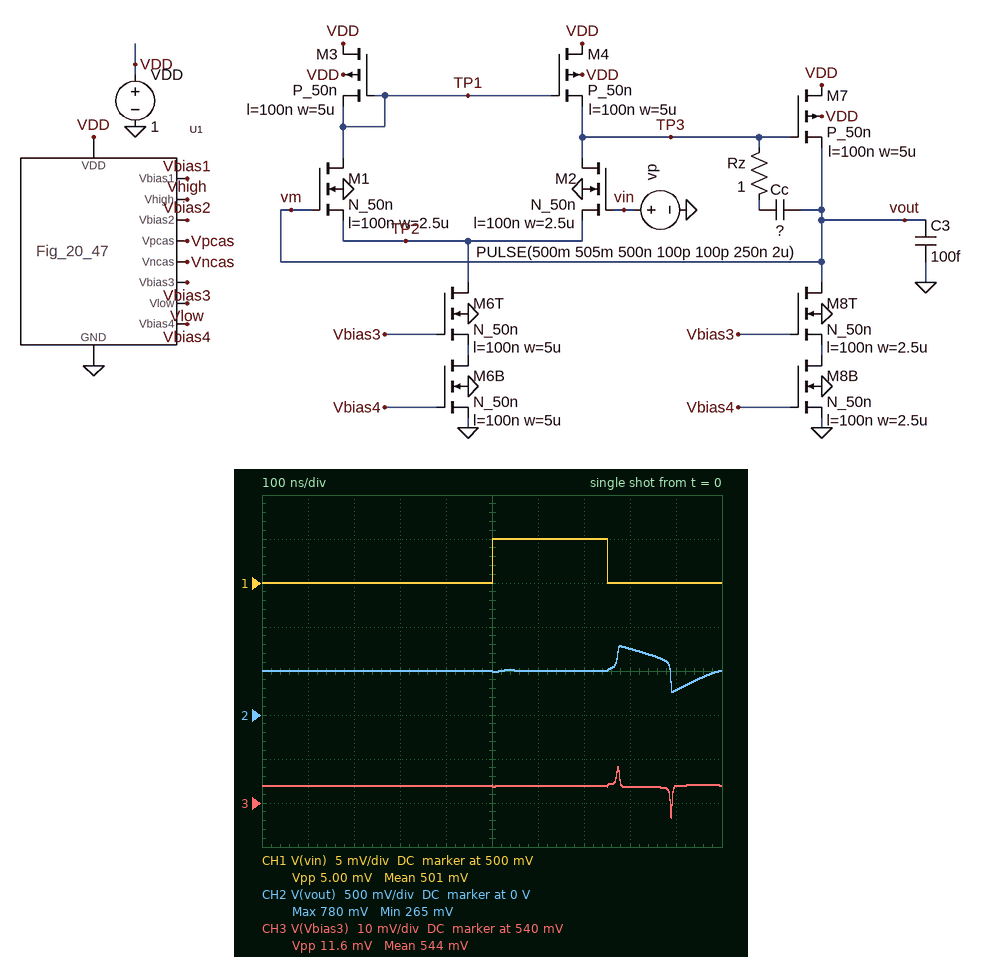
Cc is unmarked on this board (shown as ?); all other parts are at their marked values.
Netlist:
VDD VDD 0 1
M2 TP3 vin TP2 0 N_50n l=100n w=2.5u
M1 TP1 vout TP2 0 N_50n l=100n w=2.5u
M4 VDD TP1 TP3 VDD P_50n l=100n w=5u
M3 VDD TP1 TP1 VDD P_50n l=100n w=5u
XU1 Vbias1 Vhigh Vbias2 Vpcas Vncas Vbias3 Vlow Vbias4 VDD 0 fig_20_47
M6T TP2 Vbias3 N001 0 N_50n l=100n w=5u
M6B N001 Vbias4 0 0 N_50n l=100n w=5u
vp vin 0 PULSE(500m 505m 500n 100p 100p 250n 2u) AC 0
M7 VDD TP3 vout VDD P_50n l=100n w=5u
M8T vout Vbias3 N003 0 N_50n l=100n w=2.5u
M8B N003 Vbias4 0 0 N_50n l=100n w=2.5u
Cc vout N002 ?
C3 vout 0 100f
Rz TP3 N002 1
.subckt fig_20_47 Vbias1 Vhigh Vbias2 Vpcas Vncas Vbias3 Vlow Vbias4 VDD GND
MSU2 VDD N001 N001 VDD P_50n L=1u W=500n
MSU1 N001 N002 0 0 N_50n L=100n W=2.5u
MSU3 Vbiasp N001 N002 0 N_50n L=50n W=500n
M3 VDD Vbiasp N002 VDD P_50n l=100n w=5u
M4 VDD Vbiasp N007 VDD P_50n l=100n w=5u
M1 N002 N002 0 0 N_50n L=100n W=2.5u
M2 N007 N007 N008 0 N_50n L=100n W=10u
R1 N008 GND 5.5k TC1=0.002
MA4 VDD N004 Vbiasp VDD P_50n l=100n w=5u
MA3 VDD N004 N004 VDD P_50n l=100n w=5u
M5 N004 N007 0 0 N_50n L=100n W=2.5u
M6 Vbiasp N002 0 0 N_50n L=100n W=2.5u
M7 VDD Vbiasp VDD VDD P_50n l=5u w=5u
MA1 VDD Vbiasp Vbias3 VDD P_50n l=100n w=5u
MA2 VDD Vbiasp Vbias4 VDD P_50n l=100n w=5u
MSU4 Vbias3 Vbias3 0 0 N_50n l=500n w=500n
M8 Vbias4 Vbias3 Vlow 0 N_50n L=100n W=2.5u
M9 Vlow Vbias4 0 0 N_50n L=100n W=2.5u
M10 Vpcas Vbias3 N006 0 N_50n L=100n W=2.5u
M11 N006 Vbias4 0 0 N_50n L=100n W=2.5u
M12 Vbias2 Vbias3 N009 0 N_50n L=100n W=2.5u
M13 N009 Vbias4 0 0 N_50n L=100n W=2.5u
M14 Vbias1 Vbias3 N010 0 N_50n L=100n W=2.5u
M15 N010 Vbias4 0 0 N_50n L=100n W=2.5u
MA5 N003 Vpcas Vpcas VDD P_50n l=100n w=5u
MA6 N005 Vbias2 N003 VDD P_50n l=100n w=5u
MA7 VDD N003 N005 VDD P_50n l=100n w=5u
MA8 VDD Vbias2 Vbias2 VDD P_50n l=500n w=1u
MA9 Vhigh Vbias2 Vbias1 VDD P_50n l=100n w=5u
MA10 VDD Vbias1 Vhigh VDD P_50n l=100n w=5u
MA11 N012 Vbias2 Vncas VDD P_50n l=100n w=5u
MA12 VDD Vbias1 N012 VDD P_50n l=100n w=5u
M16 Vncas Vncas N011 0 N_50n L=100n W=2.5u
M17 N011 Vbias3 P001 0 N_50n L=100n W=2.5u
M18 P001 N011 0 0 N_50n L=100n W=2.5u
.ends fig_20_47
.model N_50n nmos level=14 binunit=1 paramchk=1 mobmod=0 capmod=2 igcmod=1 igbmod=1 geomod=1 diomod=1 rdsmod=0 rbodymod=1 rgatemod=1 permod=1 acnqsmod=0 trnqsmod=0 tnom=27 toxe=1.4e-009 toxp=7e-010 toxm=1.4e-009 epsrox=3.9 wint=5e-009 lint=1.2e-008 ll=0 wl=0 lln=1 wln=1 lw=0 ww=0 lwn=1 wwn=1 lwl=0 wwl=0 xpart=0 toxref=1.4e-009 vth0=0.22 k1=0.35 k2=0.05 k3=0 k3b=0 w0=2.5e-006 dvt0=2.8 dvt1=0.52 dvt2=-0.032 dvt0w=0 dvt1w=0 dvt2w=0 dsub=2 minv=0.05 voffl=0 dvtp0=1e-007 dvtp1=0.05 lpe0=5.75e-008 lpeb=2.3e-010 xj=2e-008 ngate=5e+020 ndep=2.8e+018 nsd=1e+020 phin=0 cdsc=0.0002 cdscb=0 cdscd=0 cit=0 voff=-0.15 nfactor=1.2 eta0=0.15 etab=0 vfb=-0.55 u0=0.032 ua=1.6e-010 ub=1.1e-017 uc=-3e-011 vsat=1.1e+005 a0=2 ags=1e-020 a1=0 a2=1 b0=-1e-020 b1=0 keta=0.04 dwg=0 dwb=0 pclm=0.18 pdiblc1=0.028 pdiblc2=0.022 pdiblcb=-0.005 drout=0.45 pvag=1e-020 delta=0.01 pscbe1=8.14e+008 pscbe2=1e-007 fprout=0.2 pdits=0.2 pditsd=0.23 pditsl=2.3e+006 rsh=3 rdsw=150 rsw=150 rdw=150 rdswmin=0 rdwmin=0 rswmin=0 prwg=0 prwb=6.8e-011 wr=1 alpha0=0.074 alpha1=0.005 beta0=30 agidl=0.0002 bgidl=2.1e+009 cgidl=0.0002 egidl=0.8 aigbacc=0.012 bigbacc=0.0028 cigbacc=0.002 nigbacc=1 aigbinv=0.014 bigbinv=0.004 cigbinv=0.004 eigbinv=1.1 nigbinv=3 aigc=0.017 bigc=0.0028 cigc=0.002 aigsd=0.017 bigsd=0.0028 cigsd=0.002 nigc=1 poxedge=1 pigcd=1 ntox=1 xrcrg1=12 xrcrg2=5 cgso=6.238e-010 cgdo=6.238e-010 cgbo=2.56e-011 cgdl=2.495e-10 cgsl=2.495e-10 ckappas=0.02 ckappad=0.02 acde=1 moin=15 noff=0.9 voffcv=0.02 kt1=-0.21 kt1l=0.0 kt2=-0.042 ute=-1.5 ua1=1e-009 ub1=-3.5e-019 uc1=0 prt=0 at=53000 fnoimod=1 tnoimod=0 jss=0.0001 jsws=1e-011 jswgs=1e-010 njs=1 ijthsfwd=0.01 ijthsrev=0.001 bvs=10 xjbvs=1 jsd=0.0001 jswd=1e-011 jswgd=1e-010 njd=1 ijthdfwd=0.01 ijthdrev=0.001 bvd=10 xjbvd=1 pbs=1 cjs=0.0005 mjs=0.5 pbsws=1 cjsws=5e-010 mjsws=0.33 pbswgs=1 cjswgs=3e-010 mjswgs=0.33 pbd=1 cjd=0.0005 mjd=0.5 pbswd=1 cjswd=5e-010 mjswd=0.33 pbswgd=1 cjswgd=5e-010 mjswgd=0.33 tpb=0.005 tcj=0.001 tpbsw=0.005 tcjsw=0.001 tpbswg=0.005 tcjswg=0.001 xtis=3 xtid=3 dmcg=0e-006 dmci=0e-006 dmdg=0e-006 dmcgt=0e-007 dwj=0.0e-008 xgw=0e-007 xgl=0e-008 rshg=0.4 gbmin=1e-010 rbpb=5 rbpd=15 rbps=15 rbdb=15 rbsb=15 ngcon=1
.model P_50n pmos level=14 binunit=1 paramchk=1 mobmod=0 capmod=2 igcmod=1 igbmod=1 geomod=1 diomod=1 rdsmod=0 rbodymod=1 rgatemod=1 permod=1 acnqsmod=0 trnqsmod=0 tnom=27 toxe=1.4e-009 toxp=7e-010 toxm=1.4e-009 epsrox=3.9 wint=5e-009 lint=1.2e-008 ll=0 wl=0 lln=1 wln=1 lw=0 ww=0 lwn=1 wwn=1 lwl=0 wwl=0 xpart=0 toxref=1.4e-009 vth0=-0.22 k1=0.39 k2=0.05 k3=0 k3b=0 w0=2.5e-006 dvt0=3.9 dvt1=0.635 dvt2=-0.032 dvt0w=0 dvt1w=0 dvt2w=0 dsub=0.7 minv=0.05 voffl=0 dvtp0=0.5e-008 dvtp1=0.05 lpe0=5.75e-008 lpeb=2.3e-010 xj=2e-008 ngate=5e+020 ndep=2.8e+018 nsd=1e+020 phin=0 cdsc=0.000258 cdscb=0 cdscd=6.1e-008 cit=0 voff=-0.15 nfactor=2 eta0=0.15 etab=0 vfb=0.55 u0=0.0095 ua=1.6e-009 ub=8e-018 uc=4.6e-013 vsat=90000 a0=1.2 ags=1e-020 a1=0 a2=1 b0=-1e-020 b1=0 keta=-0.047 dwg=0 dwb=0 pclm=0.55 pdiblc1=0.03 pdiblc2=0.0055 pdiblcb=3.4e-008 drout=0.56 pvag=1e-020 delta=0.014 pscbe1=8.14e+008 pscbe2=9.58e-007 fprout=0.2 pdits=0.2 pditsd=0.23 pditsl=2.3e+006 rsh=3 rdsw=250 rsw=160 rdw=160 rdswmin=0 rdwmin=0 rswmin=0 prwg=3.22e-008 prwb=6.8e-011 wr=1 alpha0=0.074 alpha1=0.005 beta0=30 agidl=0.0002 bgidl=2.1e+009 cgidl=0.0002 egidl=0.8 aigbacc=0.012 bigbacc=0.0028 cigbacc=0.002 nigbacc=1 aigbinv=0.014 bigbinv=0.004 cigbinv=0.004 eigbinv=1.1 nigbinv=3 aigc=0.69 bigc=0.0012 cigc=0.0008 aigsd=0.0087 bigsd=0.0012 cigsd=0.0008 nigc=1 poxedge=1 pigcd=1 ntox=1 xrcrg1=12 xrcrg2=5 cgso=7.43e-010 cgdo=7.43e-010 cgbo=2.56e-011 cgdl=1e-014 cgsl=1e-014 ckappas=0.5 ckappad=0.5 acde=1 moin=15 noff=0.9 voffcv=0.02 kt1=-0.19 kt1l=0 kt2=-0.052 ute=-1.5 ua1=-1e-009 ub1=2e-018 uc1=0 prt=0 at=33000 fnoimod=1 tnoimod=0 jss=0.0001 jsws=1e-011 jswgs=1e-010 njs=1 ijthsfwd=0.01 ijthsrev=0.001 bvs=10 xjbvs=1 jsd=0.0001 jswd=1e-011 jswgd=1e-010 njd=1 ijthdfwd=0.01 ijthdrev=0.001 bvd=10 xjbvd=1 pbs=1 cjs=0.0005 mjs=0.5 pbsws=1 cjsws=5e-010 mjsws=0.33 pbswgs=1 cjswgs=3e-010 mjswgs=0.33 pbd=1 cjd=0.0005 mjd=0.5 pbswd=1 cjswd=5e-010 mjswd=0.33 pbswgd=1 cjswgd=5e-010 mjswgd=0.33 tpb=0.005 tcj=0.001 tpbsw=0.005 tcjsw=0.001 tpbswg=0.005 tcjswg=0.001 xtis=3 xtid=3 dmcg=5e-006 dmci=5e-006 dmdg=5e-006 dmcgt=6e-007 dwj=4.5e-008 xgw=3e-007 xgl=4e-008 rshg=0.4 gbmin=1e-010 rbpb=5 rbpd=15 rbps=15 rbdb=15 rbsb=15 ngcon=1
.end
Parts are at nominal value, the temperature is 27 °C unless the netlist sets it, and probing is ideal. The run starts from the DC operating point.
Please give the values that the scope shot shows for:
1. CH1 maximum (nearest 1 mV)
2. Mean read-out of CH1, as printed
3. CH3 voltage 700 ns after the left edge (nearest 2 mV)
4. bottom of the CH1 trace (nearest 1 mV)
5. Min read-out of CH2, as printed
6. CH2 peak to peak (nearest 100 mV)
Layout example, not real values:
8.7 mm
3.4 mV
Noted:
505 mV
501 mV
544 mV
500 mV
265 mV
500 mV
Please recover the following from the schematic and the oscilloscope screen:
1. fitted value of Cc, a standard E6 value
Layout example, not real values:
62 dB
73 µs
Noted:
6.8 pF
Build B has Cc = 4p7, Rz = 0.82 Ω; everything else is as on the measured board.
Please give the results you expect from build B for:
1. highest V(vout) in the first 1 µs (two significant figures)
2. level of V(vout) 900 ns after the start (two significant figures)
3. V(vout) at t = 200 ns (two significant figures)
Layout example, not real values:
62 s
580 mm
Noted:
530 mV
500 mV
500 mV
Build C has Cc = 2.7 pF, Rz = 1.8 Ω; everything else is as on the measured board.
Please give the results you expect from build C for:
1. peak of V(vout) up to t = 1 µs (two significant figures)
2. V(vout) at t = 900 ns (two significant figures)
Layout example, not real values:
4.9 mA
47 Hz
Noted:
520 mV
500 mV
